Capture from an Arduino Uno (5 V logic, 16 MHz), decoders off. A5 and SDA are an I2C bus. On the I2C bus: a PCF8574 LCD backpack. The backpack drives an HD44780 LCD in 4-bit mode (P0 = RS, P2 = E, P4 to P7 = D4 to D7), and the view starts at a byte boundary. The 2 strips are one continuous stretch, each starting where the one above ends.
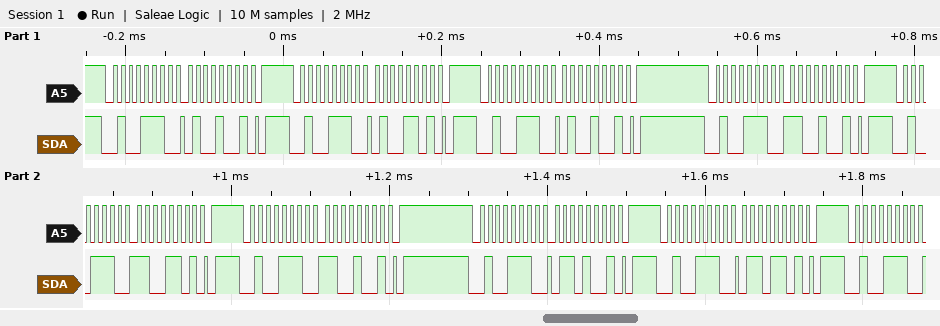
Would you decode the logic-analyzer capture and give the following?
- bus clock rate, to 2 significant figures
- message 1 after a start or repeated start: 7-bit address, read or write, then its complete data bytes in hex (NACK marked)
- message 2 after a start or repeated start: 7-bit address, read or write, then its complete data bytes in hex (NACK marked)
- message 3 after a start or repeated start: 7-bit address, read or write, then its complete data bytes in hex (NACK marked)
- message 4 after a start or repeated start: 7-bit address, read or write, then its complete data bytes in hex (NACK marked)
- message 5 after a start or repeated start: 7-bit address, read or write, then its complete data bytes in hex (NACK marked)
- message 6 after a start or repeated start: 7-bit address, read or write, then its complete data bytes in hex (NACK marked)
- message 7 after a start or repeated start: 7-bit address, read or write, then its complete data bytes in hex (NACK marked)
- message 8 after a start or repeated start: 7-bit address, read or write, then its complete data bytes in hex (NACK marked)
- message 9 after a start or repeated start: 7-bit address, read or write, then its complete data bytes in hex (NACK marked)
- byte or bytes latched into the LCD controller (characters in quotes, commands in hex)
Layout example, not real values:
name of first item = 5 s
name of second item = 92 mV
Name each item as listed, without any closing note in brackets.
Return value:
bus clock rate, to 2 significant figures = 100 kHz
message 1 after a start or repeated start: 7-bit address, read or write, then its complete data bytes in hex = 0x27 write: 49
message 2 after a start or repeated start: 7-bit address, read or write, then its complete data bytes in hex = 0x27 write: 4D
message 3 after a start or repeated start: 7-bit address, read or write, then its complete data bytes in hex = 0x27 write: 49
message 4 after a start or repeated start: 7-bit address, read or write, then its complete data bytes in hex = 0x27 write: C9
message 5 after a start or repeated start: 7-bit address, read or write, then its complete data bytes in hex = 0x27 write: CD
message 6 after a start or repeated start: 7-bit address, read or write, then its complete data bytes in hex = 0x27 write: C9
message 7 after a start or repeated start: 7-bit address, read or write, then its complete data bytes in hex = 0x27 write: 69
message 8 after a start or repeated start: 7-bit address, read or write, then its complete data bytes in hex = 0x27 write: 6D
message 9 after a start or repeated start: 7-bit address, read or write, then its complete data bytes in hex = 0x27 write
byte or bytes latched into the LCD controller = 'L'
